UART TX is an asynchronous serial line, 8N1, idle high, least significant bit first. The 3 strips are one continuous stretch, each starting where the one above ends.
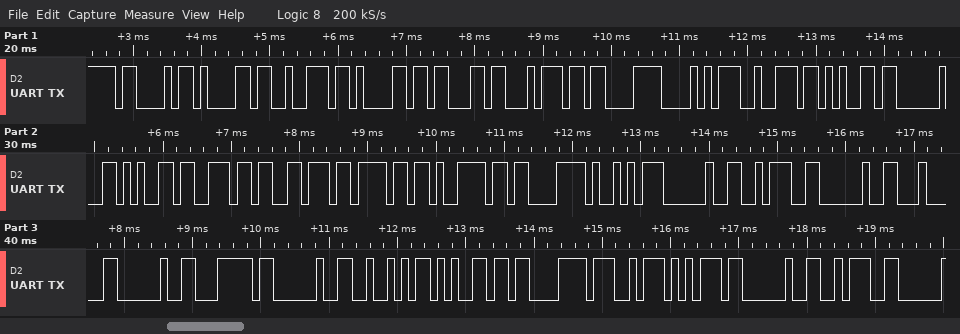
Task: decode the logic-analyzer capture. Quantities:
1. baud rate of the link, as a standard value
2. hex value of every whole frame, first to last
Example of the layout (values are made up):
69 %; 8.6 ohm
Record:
9600 baud; 43 61 72 61 63 74 C3 A8 72 65 20 65 6E 76 6F 79 C3 A9 20 3A 20 04 20 7C 20 52 65 C3 A7 75 20 3A
